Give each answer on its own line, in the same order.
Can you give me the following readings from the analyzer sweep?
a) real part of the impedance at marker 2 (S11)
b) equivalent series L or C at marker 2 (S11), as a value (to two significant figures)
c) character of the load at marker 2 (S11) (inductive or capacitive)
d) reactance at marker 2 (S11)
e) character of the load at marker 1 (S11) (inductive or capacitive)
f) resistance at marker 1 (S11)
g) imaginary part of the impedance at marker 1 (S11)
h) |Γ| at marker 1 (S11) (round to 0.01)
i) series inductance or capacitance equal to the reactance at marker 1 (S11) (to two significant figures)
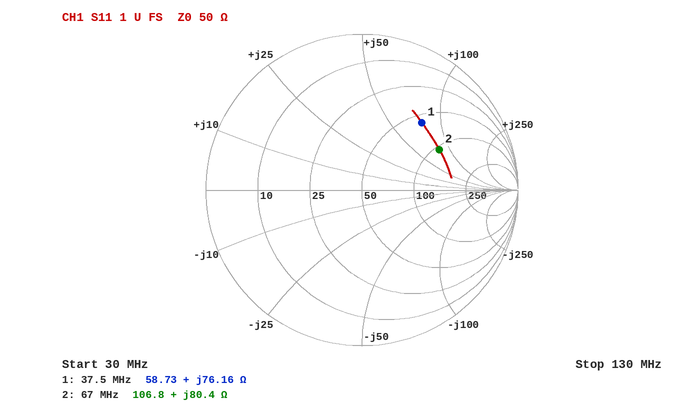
106.8 Ω
190 nH
inductive
+80.4 Ω
inductive
58.73 Ω
+76.16 Ω
0.58
320 nH
